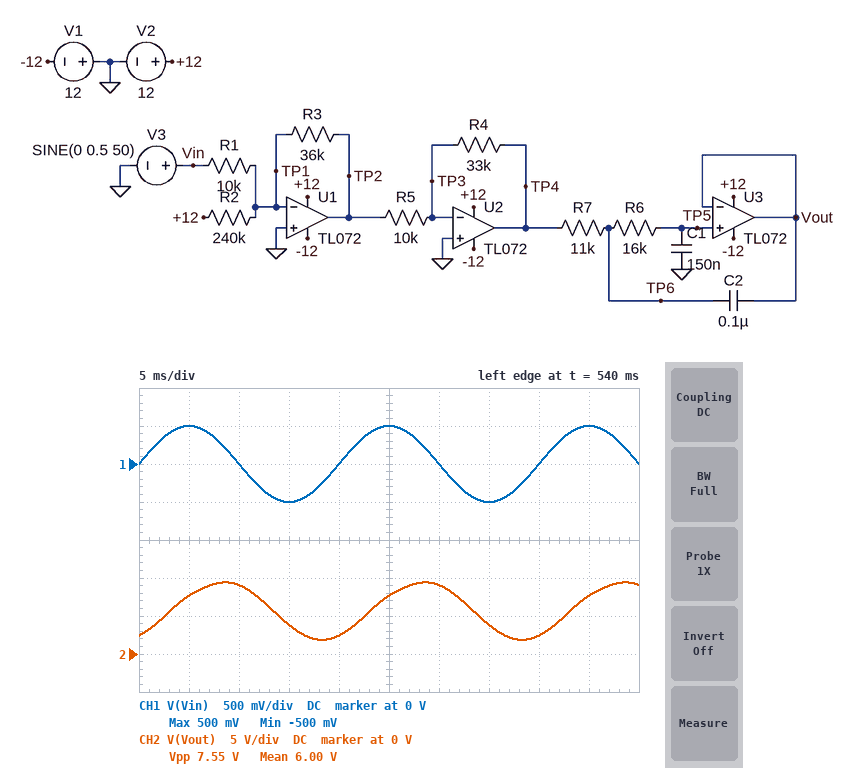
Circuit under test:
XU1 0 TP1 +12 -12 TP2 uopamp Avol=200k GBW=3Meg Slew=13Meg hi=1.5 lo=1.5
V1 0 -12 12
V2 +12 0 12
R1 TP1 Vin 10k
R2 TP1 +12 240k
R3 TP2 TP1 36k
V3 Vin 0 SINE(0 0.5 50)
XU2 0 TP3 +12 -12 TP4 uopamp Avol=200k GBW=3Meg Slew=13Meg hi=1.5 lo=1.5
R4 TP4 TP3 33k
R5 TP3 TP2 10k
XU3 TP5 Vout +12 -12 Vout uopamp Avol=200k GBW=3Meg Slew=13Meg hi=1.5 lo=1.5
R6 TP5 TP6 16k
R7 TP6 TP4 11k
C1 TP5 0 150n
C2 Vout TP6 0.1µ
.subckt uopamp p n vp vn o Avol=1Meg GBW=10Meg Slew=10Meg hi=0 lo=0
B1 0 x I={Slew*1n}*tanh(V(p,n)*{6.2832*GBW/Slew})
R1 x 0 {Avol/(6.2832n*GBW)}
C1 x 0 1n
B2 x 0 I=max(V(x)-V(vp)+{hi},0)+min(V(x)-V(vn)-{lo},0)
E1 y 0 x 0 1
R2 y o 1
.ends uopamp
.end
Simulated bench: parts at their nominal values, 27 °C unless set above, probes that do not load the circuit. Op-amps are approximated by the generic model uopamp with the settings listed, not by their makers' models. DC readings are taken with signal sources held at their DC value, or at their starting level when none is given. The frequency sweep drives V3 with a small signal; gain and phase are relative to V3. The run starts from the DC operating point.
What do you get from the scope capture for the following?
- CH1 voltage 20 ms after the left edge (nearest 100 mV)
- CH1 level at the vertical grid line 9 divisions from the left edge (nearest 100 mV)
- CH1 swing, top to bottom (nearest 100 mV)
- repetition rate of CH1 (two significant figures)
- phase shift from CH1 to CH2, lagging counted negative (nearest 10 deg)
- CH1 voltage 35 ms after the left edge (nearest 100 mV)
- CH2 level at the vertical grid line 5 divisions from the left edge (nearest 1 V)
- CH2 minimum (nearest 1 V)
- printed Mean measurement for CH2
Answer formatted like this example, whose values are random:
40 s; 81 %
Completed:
0 V; 500 mV; 1.0 V; 50 Hz; -60 deg; -500 mV; 8 V; 2 V; 6.00 V
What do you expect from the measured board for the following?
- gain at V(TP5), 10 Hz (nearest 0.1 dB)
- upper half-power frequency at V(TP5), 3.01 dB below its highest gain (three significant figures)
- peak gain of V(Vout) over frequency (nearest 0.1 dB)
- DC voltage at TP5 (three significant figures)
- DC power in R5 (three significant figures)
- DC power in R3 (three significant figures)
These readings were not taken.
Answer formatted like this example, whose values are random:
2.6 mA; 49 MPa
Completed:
21.3 dB; 46.5 Hz; 21.5 dB; 5.94 V; 324 µW; 90.0 µW
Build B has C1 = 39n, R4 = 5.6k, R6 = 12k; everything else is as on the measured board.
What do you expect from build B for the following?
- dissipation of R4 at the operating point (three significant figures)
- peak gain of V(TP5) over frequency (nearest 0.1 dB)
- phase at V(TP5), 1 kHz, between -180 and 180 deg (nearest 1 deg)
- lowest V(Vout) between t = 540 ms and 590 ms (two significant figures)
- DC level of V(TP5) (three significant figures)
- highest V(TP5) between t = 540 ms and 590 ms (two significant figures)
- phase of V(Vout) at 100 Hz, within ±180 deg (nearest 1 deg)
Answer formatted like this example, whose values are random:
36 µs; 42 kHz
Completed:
181 µW; 6.3 dB; -164 deg; -10 mV; 1.01 V; 2.0 V; -35 deg
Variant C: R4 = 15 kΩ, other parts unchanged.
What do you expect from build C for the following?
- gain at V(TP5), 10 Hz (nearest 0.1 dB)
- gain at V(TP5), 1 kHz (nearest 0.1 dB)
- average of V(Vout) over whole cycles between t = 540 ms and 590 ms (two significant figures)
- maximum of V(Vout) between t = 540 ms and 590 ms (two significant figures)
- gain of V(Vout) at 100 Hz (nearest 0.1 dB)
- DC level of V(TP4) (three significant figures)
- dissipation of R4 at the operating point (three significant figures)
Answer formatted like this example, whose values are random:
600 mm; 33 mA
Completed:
14.5 dB; -25.9 dB; 2.7 V; 4.5 V; 6.5 dB; 2.70 V; 486 µW
